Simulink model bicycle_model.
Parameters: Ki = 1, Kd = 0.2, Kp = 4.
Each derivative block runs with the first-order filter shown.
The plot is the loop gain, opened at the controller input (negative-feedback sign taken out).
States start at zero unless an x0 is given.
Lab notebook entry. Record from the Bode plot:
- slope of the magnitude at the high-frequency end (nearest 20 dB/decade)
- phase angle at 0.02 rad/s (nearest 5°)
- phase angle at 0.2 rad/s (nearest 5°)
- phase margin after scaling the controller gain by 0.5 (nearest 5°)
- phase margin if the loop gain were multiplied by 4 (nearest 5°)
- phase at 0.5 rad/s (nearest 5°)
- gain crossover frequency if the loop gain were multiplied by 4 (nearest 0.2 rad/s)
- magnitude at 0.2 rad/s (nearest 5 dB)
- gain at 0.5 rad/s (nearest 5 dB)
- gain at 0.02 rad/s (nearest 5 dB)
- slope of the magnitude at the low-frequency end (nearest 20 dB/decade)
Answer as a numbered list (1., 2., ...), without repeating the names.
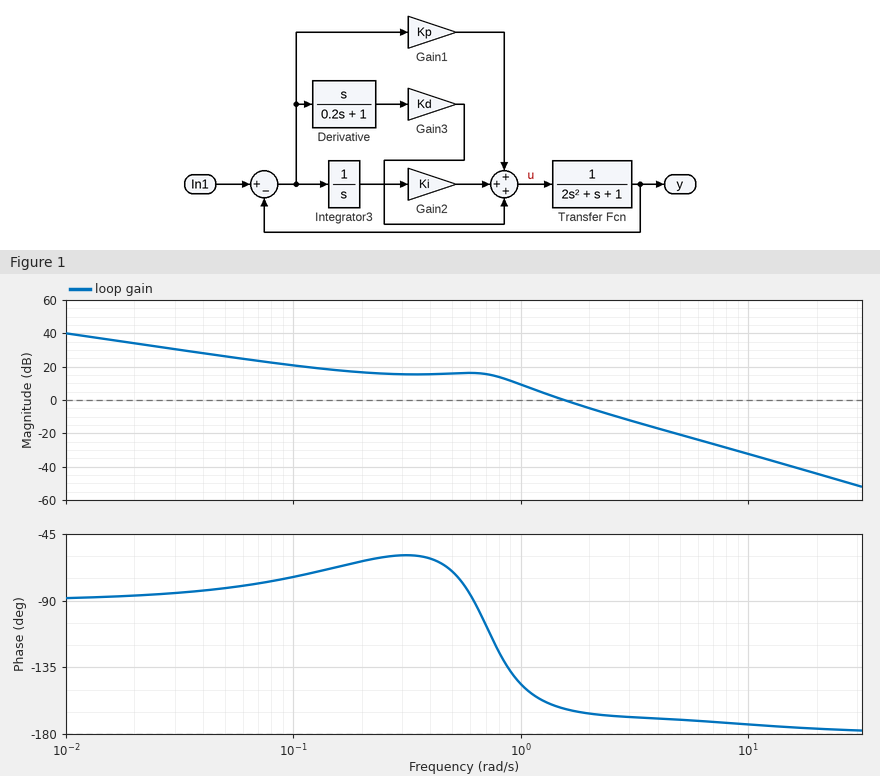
1. -40 dB/decade
2. -85°
3. -65°
4. 25°
5. 10°
6. -70°
7. 3.0 rad/s
8. 15 dB
9. 15 dB
10. 35 dB
11. -20 dB/decade
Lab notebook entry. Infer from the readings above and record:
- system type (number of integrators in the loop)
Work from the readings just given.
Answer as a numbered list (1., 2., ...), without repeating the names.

1. 1
